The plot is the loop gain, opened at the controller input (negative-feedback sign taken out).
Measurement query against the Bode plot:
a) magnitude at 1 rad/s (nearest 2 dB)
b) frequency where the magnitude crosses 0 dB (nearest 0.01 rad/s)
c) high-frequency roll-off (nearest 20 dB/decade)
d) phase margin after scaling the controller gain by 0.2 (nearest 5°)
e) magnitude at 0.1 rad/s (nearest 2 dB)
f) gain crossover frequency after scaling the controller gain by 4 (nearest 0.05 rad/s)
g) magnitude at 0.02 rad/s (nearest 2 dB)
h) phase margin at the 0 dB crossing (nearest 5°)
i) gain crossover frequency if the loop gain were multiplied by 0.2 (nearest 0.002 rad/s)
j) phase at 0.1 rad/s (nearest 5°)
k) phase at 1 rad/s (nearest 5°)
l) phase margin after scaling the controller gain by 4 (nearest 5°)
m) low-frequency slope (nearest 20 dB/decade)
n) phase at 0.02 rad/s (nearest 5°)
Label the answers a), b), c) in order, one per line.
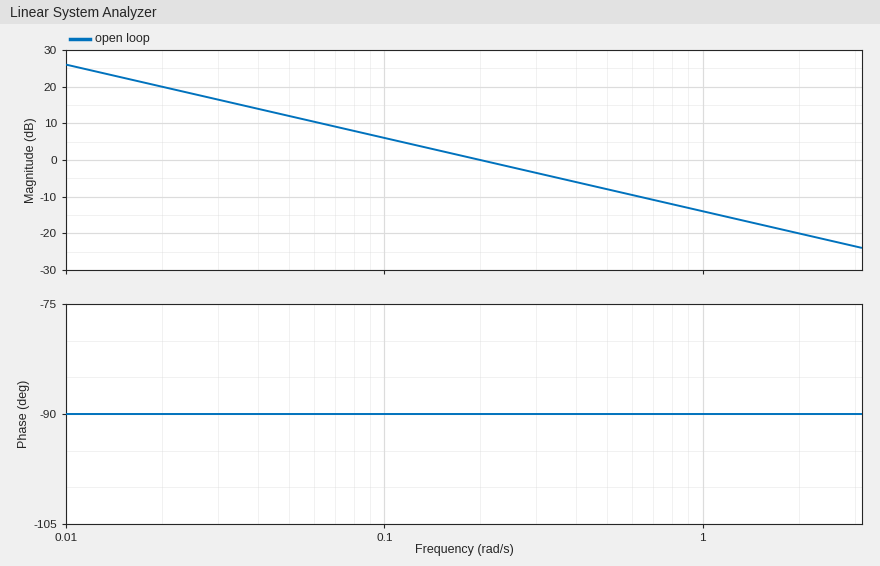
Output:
a) -14 dB
b) 0.20 rad/s
c) -20 dB/decade
d) 90°
e) 6 dB
f) 0.80 rad/s
g) 20 dB
h) 90°
i) 0.040 rad/s
j) -90°
k) -90°
l) 90°
m) -20 dB/decade
n) -90°
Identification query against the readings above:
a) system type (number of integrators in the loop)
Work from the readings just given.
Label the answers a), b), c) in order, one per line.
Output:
a) 1
